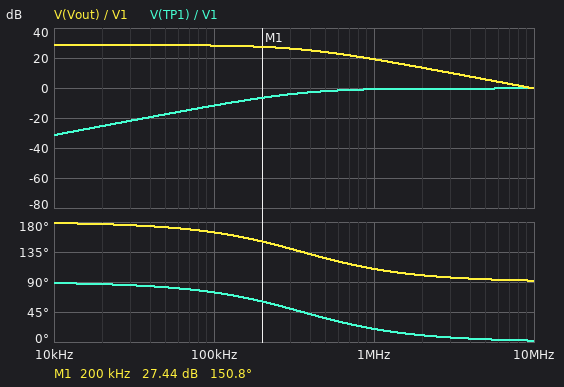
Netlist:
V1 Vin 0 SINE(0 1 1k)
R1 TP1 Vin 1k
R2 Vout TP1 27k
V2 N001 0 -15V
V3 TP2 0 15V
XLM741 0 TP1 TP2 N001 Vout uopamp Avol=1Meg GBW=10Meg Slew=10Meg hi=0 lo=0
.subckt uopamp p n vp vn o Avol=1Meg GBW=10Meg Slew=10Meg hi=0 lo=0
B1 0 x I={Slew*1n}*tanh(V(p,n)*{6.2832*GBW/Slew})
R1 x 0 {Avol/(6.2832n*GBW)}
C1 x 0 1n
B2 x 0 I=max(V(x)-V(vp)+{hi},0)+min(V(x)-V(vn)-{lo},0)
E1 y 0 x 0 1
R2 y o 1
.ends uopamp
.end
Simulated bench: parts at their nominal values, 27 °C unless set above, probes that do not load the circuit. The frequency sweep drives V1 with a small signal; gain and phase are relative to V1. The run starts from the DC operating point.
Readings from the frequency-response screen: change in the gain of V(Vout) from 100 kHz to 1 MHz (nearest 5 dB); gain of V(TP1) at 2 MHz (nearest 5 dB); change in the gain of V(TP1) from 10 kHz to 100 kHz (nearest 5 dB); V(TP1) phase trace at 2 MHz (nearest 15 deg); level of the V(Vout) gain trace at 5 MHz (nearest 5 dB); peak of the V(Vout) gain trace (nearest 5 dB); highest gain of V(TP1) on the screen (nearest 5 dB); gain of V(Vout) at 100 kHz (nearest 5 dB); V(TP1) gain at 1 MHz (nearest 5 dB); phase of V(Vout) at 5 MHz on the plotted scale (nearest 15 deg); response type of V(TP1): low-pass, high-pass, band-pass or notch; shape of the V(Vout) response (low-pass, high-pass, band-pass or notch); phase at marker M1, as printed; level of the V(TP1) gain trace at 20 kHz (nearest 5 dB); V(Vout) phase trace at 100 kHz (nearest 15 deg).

-10 dB
0 dB
20 dB
15 deg
5 dB
30 dB
0 dB
30 dB
0 dB
90 deg
high-pass
low-pass
150.8 deg
-25 dB
165 deg
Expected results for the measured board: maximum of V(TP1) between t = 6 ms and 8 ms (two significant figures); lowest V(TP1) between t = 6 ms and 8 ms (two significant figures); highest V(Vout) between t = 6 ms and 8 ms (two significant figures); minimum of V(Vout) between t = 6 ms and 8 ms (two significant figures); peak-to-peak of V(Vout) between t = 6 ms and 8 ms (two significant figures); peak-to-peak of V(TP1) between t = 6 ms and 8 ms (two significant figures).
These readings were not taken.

430 mV
-430 mV
15 V
-15 V
30 V
860 mV
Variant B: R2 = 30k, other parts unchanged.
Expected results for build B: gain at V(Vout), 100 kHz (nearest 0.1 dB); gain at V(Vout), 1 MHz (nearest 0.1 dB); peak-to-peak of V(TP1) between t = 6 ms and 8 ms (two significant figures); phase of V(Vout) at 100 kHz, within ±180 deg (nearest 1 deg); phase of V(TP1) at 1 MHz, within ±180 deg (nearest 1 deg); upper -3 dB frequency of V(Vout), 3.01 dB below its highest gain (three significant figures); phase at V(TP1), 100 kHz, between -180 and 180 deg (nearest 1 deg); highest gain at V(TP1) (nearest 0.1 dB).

29.1 dB
19.3 dB
970 mV
163 deg
18 deg
323 kHz
73 deg
-0.3 dB
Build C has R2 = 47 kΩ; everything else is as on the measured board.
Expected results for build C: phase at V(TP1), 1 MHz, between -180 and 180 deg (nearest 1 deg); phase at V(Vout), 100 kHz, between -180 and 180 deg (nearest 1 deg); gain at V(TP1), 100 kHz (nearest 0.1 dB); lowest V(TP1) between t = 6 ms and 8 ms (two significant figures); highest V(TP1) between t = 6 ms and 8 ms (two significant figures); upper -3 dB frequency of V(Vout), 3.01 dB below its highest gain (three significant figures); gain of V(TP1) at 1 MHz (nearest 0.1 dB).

12 deg
154 deg
-7.5 dB
-670 mV
670 mV
208 kHz
-0.4 dB
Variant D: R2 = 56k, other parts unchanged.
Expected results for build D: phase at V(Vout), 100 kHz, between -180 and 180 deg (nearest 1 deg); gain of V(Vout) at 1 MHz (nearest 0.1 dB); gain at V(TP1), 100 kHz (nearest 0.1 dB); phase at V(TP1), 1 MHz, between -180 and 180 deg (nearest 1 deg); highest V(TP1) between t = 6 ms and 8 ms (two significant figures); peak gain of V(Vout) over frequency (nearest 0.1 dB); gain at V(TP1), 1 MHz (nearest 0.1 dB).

150 deg
19.7 dB
-6.3 dB
10 deg
720 mV
35.0 dB
-0.3 dB
